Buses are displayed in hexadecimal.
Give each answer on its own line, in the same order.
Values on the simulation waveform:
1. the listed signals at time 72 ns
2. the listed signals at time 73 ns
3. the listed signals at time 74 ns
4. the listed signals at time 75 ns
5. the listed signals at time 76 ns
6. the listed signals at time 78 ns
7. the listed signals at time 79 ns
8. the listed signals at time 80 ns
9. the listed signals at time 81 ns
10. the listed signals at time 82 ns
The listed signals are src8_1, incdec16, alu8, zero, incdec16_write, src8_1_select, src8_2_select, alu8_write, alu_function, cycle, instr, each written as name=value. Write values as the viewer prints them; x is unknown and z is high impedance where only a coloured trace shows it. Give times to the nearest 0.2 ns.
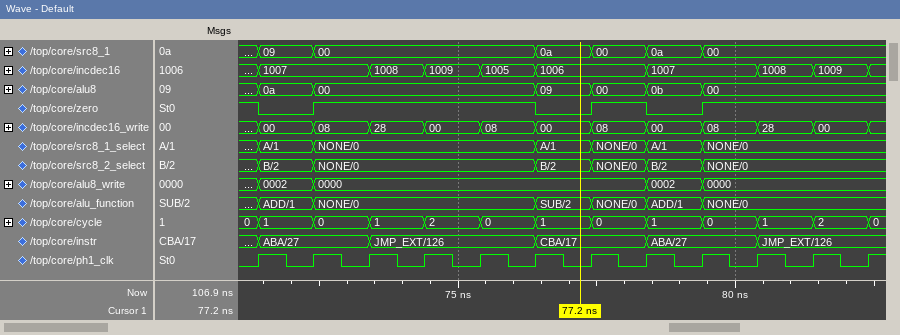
src8_1=09, incdec16=1007, alu8=0a, zero=0, incdec16_write=00, src8_1_select=A/1, src8_2_select=B/2, alu8_write=0002, alu_function=ADD/1, cycle=1, instr=ABA/27
src8_1=00, incdec16=1007, alu8=00, zero=1, incdec16_write=08, src8_1_select=NONE/0, src8_2_select=NONE/0, alu8_write=0000, alu_function=NONE/0, cycle=0, instr=ABA/27
src8_1=00, incdec16=1008, alu8=00, zero=1, incdec16_write=28, src8_1_select=NONE/0, src8_2_select=NONE/0, alu8_write=0000, alu_function=NONE/0, cycle=1, instr=JMP_EXT/126
src8_1=00, incdec16=1009, alu8=00, zero=1, incdec16_write=00, src8_1_select=NONE/0, src8_2_select=NONE/0, alu8_write=0000, alu_function=NONE/0, cycle=2, instr=JMP_EXT/126
src8_1=00, incdec16=1005, alu8=00, zero=1, incdec16_write=08, src8_1_select=NONE/0, src8_2_select=NONE/0, alu8_write=0000, alu_function=NONE/0, cycle=0, instr=JMP_EXT/126
src8_1=00, incdec16=1006, alu8=00, zero=1, incdec16_write=08, src8_1_select=NONE/0, src8_2_select=NONE/0, alu8_write=0000, alu_function=NONE/0, cycle=0, instr=CBA/17
src8_1=0a, incdec16=1007, alu8=0b, zero=0, incdec16_write=00, src8_1_select=A/1, src8_2_select=B/2, alu8_write=0002, alu_function=ADD/1, cycle=1, instr=ABA/27
src8_1=00, incdec16=1007, alu8=00, zero=1, incdec16_write=08, src8_1_select=NONE/0, src8_2_select=NONE/0, alu8_write=0000, alu_function=NONE/0, cycle=0, instr=ABA/27
src8_1=00, incdec16=1008, alu8=00, zero=1, incdec16_write=28, src8_1_select=NONE/0, src8_2_select=NONE/0, alu8_write=0000, alu_function=NONE/0, cycle=1, instr=JMP_EXT/126
src8_1=00, incdec16=1009, alu8=00, zero=1, incdec16_write=00, src8_1_select=NONE/0, src8_2_select=NONE/0, alu8_write=0000, alu_function=NONE/0, cycle=2, instr=JMP_EXT/126
